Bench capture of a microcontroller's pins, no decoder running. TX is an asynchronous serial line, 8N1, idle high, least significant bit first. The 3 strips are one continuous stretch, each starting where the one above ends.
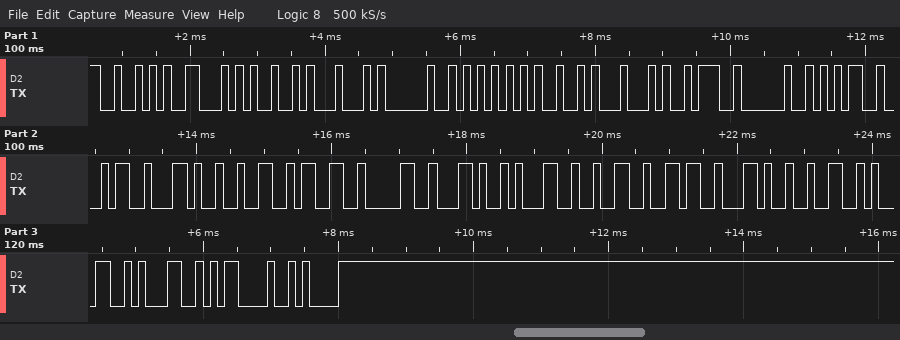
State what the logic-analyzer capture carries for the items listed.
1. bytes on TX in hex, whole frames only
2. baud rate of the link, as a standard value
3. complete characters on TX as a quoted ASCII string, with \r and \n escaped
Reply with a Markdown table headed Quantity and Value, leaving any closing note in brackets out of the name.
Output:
| Quantity | Value |
|---|---|
| bytes on TX in hex, whole frames only | 52 46 49 44 20 55 49 44 3A 20 35 34 2C 32 33 30 2C 31 32 36 2C 32 31 31 0D 0A |
| baud rate of the link, as a standard value | 9600 baud |
| complete characters on TX as a quoted ASCII string, with \r and \n escaped | "RFID UID: 54,230,126,211\r\n" |
